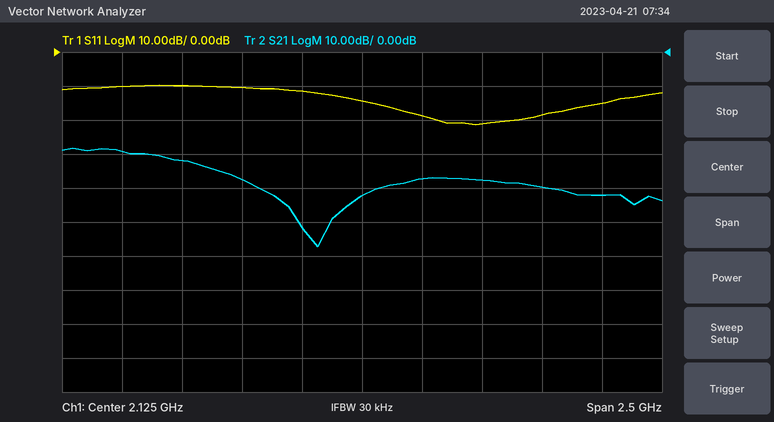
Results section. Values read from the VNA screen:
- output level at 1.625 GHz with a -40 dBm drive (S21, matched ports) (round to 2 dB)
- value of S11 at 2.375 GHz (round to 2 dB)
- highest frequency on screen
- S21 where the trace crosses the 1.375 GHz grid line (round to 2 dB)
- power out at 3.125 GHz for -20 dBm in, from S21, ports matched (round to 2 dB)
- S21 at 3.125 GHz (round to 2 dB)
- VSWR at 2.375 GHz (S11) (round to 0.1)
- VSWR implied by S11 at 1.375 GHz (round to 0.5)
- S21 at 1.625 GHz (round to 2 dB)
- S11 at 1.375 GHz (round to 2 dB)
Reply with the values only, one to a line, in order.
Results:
-78 dBm
-18 dB
3.375 GHz
-32 dB
-62 dBm
-42 dB
1.3
2.0
-38 dB
-10 dB
